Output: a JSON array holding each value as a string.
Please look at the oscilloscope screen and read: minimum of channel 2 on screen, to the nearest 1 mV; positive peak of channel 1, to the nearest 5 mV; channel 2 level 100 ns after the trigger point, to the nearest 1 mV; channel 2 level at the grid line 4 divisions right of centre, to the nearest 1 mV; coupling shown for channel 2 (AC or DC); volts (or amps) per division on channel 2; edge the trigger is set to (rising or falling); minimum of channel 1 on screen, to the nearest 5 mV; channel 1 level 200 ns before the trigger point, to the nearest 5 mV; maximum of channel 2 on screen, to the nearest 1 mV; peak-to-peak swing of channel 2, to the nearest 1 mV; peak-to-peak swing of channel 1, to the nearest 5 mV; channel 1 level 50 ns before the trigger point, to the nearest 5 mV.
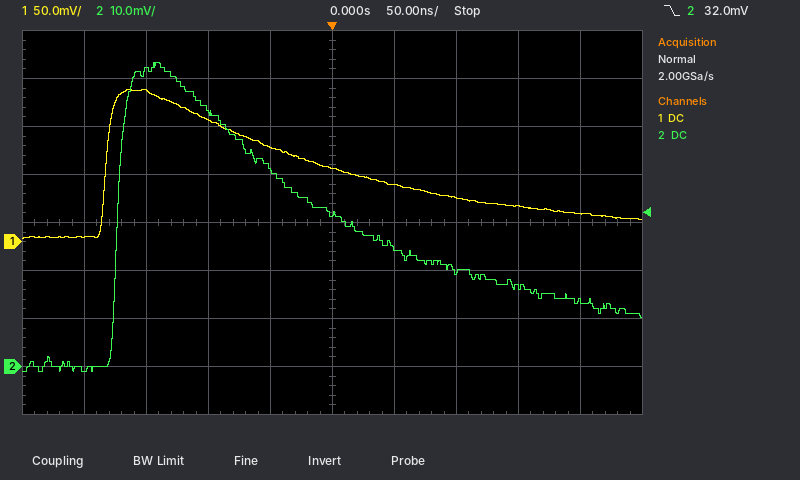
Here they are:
["-1 mV", "160 mV", "20 mV", "14 mV", "DC", "10 mV", "falling", "5 mV", "5 mV", "63 mV", "64 mV", "155 mV", "100 mV"]
